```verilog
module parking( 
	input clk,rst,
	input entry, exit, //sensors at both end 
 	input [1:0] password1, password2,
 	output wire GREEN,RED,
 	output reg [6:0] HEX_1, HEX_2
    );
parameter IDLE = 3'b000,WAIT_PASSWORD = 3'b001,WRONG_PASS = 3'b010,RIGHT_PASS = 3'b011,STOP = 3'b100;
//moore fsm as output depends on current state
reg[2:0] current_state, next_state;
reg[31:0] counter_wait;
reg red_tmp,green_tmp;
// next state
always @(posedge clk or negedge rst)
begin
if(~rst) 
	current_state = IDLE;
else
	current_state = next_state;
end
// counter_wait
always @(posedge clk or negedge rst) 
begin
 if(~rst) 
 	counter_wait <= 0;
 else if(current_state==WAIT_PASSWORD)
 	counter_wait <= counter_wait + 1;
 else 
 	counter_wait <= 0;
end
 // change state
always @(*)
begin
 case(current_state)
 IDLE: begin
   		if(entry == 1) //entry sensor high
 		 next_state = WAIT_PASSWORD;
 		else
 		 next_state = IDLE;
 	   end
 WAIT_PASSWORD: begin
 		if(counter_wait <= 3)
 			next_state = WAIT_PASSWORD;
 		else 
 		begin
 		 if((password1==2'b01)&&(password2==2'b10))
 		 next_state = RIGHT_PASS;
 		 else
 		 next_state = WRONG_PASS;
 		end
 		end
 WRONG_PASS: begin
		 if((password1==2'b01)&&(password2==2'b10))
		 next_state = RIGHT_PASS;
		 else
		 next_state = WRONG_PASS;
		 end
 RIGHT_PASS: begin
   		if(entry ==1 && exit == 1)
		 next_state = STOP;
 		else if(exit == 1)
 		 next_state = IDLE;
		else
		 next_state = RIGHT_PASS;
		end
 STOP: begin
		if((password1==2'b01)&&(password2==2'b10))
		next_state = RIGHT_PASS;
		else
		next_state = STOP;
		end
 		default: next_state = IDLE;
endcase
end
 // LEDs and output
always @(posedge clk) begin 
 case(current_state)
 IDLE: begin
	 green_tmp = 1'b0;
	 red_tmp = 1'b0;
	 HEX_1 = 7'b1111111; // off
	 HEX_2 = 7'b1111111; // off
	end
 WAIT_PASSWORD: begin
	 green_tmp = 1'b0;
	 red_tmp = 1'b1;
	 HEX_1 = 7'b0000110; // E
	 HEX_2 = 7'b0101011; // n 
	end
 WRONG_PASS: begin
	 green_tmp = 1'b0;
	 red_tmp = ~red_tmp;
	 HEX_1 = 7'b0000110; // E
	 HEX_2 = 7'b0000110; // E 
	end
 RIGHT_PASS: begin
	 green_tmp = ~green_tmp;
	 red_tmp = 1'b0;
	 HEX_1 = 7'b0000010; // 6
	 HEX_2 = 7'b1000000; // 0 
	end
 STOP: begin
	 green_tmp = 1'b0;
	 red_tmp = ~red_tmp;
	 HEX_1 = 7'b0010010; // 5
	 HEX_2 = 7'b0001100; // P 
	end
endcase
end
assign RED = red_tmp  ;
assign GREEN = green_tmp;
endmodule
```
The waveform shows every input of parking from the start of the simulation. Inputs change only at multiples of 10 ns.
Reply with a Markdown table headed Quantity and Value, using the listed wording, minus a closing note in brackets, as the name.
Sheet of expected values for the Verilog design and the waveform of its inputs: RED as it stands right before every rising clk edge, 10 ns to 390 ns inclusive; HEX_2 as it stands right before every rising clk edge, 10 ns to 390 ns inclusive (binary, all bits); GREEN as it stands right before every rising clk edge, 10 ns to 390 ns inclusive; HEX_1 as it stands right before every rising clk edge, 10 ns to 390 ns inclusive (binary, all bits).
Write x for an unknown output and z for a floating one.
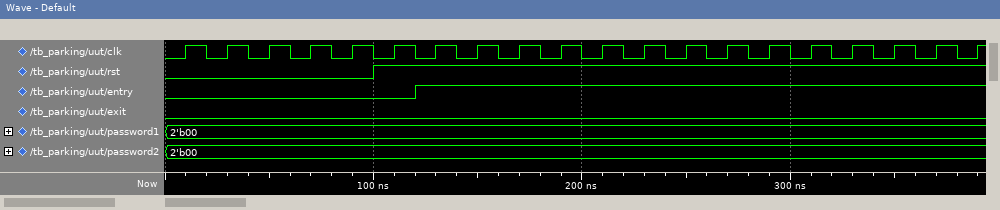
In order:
| Quantity | Value |
|---|---|
| RED as it stands right before every rising clk edge, 10 ns to 390 ns inclusive | x 0 0 0 0 0 0 1 1 1 1 0 1 0 1 0 1 0 1 0 |
| HEX_2 as it stands right before every rising clk edge, 10 ns to 390 ns inclusive | x, 1111111, 1111111, 1111111, 1111111, 1111111, 1111111, 0101011, 0101011, 0101011, 0101011, 0000110, 0000110, 0000110, 0000110, 0000110, 0000110, 0000110, 0000110, 0000110 |
| GREEN as it stands right before every rising clk edge, 10 ns to 390 ns inclusive | x 0 0 0 0 0 0 0 0 0 0 0 0 0 0 0 0 0 0 0 |
| HEX_1 as it stands right before every rising clk edge, 10 ns to 390 ns inclusive | x, 1111111, 1111111, 1111111, 1111111, 1111111, 1111111, 0000110, 0000110, 0000110, 0000110, 0000110, 0000110, 0000110, 0000110, 0000110, 0000110, 0000110, 0000110, 0000110 |
